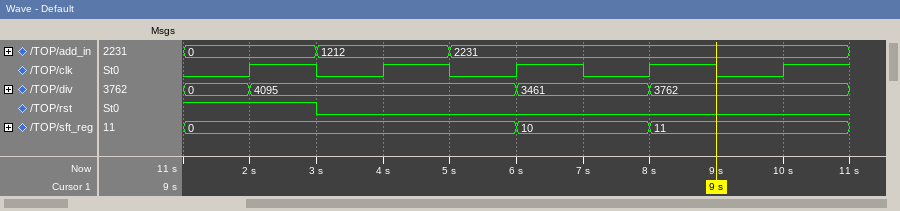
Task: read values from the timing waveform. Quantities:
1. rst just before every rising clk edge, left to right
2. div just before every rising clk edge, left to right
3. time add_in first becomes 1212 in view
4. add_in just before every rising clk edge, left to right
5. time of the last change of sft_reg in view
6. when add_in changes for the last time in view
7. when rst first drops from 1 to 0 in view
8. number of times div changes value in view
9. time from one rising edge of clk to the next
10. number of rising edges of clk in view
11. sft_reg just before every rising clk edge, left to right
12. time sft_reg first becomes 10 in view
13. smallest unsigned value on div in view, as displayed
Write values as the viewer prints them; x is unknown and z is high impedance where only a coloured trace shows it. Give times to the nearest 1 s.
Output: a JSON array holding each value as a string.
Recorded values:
["1 0 0 0 0", "0, 4095, 4095, 3461, 3762", "3 s", "0, 1212, 2231, 2231, 2231", "8 s", "5 s", "3 s", "3", "2 s", "5", "0, 0, 0, 10, 11", "6 s", "0"]
